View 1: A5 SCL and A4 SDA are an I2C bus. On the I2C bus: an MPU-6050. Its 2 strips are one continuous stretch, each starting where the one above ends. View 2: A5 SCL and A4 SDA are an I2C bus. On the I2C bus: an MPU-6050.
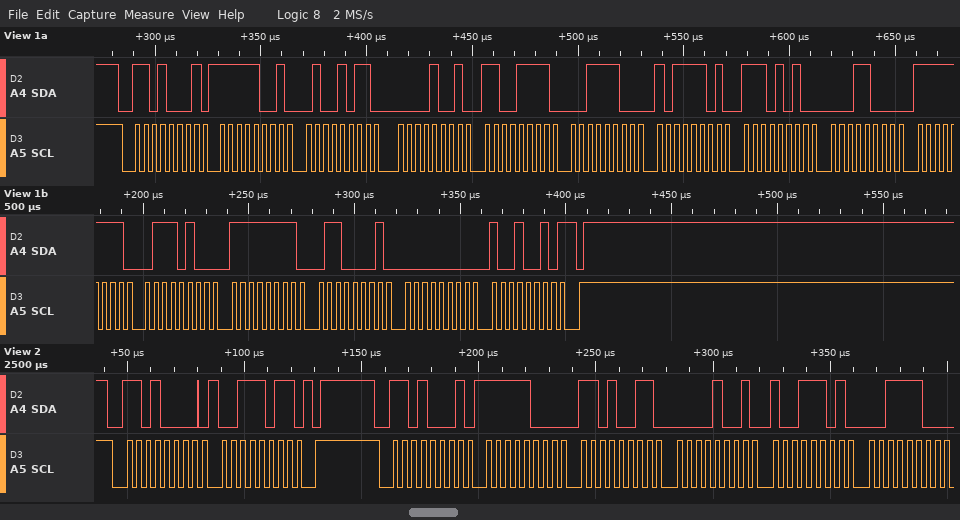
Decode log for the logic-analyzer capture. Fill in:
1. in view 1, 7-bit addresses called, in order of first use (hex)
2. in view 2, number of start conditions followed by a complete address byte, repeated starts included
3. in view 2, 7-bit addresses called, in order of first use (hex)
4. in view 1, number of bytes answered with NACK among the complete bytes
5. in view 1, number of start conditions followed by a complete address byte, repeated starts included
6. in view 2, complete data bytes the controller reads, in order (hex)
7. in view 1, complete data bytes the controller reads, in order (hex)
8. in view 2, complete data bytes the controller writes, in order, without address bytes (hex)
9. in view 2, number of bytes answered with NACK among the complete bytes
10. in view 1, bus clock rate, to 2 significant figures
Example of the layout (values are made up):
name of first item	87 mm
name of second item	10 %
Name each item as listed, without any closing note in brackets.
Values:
in view 1, 7-bit addresses called, in order of first use	0x68
in view 2, number of start conditions followed by a complete address byte, repeated starts included	2
in view 2, 7-bit addresses called, in order of first use	0x68
in view 1, number of bytes answered with NACK among the complete bytes	1
in view 1, number of start conditions followed by a complete address byte, repeated starts included	1
in view 2, complete data bytes the controller reads, in order	F8 D3 09 9D 3C
in view 1, complete data bytes the controller reads, in order	F9 4B 09 CF 3C BD EA 18 FF 74 FF 61 00 92
in view 2, complete data bytes the controller writes, in order, without address bytes	3B
in view 2, number of bytes answered with NACK among the complete bytes	0
in view 1, bus clock rate, to 2 significant figures	250 kHz
